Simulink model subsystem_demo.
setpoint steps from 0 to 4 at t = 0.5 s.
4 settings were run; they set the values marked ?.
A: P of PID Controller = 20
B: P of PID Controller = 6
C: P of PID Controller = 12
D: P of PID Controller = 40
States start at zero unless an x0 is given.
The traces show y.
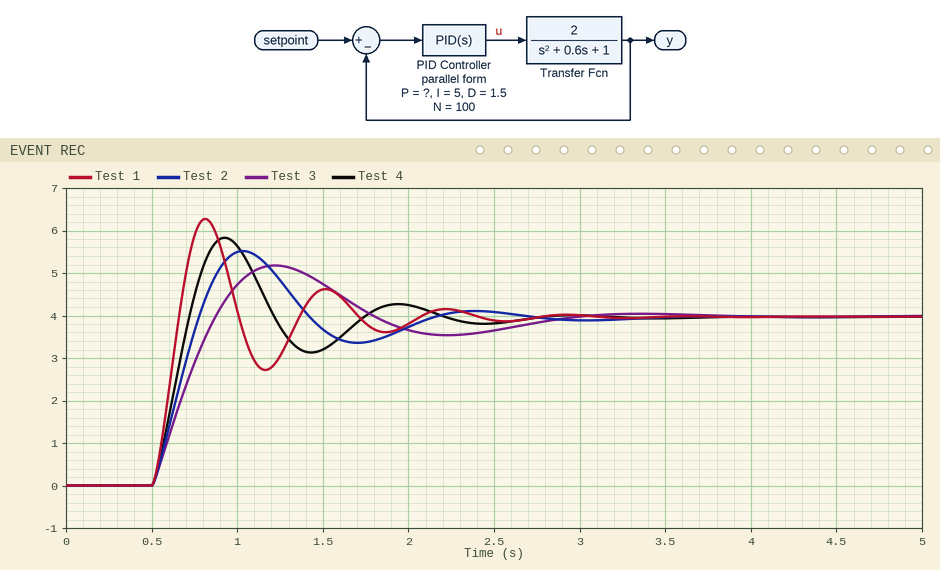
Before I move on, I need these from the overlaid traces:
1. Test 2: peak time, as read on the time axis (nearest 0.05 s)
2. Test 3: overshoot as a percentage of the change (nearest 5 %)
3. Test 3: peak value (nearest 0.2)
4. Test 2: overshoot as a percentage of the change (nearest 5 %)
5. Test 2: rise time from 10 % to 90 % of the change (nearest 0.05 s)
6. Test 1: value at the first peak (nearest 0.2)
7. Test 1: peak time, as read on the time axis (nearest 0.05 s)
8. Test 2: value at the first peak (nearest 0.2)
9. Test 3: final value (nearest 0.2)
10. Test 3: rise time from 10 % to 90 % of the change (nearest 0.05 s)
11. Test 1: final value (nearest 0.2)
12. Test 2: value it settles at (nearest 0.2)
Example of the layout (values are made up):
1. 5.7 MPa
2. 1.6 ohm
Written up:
1. 1.05 s
2. 30 %
3. 5.2
4. 40 %
5. 0.20 s
6. 6.2
7. 0.80 s
8. 5.6
9. 4.0
10. 0.30 s
11. 4.0
12. 4.0
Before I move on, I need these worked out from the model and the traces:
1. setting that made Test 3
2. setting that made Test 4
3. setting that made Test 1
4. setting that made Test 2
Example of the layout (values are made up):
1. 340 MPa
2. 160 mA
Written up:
1. B
2. A
3. D
4. C
